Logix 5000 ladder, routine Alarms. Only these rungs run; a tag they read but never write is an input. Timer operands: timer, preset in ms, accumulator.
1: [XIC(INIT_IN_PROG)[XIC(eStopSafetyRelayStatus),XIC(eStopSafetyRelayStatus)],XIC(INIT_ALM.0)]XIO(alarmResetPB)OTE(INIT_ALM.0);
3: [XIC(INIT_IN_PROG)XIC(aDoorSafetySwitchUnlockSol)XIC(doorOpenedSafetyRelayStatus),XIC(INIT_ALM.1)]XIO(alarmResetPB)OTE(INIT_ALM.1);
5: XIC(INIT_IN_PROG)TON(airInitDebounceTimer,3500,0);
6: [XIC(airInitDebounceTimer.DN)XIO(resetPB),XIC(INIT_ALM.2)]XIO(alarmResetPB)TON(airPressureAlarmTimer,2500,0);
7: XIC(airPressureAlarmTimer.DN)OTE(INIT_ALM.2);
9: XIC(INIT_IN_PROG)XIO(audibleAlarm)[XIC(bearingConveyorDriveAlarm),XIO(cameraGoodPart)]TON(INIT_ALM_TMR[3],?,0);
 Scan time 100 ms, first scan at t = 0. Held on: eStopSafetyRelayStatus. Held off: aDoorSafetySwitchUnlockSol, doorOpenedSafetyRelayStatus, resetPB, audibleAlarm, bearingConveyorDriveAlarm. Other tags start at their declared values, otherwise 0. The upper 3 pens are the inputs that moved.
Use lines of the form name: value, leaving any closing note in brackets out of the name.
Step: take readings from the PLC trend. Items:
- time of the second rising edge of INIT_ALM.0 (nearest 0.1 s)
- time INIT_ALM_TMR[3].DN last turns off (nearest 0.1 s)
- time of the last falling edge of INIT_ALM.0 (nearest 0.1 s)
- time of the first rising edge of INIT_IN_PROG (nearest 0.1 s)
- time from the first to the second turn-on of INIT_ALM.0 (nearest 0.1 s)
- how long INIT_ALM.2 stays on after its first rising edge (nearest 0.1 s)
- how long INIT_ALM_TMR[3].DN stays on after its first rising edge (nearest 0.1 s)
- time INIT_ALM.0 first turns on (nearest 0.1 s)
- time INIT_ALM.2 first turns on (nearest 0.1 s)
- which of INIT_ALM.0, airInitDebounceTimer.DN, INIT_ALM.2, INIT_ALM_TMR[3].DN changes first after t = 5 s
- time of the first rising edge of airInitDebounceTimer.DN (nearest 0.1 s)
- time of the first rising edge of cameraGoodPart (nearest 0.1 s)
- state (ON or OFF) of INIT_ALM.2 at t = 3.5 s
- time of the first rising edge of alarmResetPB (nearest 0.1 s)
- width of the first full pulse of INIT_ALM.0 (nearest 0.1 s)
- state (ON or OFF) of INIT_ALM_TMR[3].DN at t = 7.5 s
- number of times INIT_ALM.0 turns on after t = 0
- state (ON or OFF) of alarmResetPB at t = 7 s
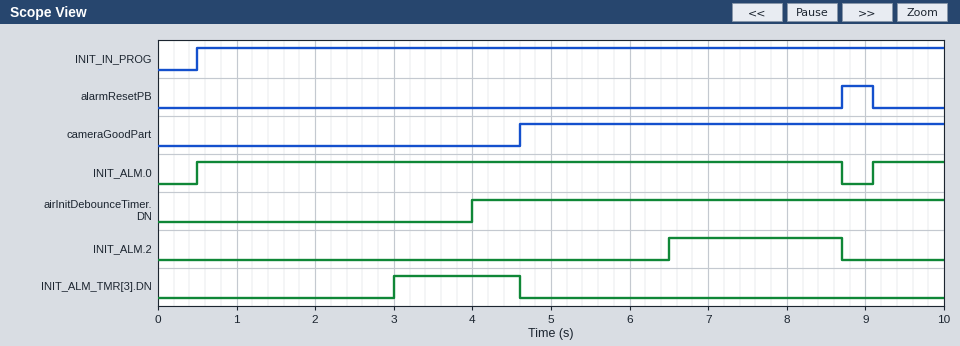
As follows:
time of the second rising edge of INIT_ALM.0: 9.1 s
time INIT_ALM_TMR[3].DN last turns off: 4.6 s
time of the last falling edge of INIT_ALM.0: 8.7 s
time of the first rising edge of INIT_IN_PROG: 0.5 s
time from the first to the second turn-on of INIT_ALM.0: 8.6 s
how long INIT_ALM.2 stays on after its first rising edge: 2.2 s
how long INIT_ALM_TMR[3].DN stays on after its first rising edge: 1.6 s
time INIT_ALM.0 first turns on: 0.5 s
time INIT_ALM.2 first turns on: 6.5 s
which of INIT_ALM.0, airInitDebounceTimer.DN, INIT_ALM.2, INIT_ALM_TMR[3].DN changes first after t = 5 s: INIT_ALM.2
time of the first rising edge of airInitDebounceTimer.DN: 4.0 s
time of the first rising edge of cameraGoodPart: 4.6 s
state (ON or OFF) of INIT_ALM.2 at t = 3.5 s: OFF
time of the first rising edge of alarmResetPB: 8.7 s
width of the first full pulse of INIT_ALM.0: 8.2 s
state (ON or OFF) of INIT_ALM_TMR[3].DN at t = 7.5 s: OFF
number of times INIT_ALM.0 turns on after t = 0: 2
state (ON or OFF) of alarmResetPB at t = 7 s: OFF
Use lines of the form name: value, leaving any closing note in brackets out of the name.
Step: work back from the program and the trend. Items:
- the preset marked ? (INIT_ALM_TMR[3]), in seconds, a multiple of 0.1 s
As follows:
the preset marked ? (INIT_ALM_TMR[3]), in seconds, a multiple of 0.1 s: 2.5 s
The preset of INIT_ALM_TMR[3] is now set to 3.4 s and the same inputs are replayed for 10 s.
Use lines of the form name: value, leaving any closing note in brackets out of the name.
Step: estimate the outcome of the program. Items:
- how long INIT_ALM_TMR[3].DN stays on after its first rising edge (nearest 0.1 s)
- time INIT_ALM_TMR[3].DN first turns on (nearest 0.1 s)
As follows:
how long INIT_ALM_TMR[3].DN stays on after its first rising edge: 0.7 s
time INIT_ALM_TMR[3].DN first turns on: 3.9 s
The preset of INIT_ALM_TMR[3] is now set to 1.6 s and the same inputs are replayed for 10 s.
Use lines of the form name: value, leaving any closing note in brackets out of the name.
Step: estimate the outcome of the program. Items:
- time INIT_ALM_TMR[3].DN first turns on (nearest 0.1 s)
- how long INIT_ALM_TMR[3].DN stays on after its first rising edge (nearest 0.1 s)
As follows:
time INIT_ALM_TMR[3].DN first turns on: 2.1 s
how long INIT_ALM_TMR[3].DN stays on after its first rising edge: 2.5 s
